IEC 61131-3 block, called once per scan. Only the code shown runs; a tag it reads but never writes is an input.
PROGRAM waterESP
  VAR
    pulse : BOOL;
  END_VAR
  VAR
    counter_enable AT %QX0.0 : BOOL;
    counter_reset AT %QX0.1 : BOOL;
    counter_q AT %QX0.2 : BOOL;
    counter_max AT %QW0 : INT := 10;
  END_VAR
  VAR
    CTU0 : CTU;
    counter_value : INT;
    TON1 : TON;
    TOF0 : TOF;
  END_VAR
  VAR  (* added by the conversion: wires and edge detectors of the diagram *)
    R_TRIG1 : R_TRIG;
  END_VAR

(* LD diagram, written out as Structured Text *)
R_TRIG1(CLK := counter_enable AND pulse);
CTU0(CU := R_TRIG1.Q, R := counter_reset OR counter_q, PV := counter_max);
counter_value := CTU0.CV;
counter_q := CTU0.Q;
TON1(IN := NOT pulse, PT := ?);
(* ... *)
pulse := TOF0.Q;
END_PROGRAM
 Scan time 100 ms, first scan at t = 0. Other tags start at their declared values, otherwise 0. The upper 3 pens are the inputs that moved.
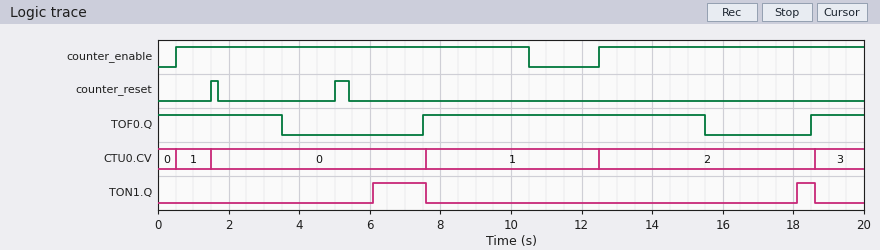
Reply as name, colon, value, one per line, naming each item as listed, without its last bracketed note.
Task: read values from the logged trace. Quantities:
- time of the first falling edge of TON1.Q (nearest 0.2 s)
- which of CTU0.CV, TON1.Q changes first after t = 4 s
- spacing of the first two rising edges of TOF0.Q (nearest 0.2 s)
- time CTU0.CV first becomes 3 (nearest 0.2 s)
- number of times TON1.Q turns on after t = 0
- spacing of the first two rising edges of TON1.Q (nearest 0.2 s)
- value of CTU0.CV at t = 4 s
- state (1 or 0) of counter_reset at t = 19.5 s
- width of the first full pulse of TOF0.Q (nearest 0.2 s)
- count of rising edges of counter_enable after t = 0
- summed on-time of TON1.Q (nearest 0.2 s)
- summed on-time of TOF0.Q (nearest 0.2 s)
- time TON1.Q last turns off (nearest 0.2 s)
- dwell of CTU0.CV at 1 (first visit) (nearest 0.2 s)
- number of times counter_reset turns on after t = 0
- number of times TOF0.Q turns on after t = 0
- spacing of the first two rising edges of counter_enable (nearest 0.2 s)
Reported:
time of the first falling edge of TON1.Q: 7.6 s
which of CTU0.CV, TON1.Q changes first after t = 4 s: TON1.Q
spacing of the first two rising edges of TOF0.Q: 11.0 s
time CTU0.CV first becomes 3: 18.6 s
number of times TON1.Q turns on after t = 0: 2
spacing of the first two rising edges of TON1.Q: 12.0 s
value of CTU0.CV at t = 4 s: 0
state (1 or 0) of counter_reset at t = 19.5 s: 0
width of the first full pulse of TOF0.Q: 8.0 s
count of rising edges of counter_enable after t = 0: 2
summed on-time of TON1.Q: 2.0 s
summed on-time of TOF0.Q: 13.0 s
time TON1.Q last turns off: 18.6 s
dwell of CTU0.CV at 1 (first visit): 1.0 s
number of times counter_reset turns on after t = 0: 2
number of times TOF0.Q turns on after t = 0: 2
spacing of the first two rising edges of counter_enable: 12.0 s
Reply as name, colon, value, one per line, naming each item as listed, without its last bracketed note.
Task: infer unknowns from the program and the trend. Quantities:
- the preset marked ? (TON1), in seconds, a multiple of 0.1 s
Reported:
the preset marked ? (TON1), in seconds, a multiple of 0.1 s: 2.5 s
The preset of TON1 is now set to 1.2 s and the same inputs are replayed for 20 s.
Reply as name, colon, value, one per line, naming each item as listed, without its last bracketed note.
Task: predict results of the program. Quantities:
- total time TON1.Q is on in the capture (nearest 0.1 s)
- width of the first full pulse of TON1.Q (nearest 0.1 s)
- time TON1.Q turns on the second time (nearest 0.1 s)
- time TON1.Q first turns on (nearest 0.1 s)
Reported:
total time TON1.Q is on in the capture: 4.6 s
width of the first full pulse of TON1.Q: 2.8 s
time TON1.Q turns on the second time: 16.8 s
time TON1.Q first turns on: 4.8 s
